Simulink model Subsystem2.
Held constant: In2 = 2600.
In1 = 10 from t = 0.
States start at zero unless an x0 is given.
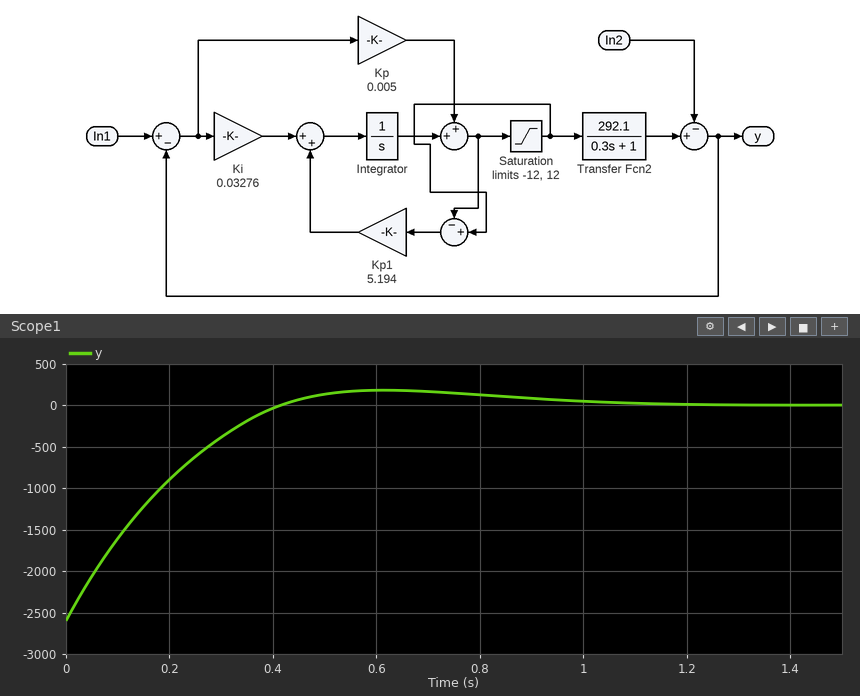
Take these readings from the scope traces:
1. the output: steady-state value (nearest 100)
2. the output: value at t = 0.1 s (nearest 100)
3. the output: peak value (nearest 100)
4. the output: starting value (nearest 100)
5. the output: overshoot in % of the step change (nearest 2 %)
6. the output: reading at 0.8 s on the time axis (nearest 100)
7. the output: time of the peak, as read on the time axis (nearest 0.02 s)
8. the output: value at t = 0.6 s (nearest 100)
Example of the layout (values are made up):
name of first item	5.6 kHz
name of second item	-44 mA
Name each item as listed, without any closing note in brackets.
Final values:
the output: steady-state value	0
the output: value at t = 0.1 s	-1600
the output: peak value	200
the output: starting value	-2600
the output: overshoot in % of the step change	6 %
the output: reading at 0.8 s on the time axis	100
the output: time of the peak, as read on the time axis	0.62 s
the output: value at t = 0.6 s	200
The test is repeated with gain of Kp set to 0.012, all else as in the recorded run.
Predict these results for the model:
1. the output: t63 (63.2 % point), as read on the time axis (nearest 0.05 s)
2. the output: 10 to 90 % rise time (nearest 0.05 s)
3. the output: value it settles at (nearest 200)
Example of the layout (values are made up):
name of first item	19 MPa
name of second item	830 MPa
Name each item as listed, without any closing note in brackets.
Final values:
the output: t63 (63.2 % point), as read on the time axis	0.20 s
the output: 10 to 90 % rise time	0.40 s
the output: value it settles at	0
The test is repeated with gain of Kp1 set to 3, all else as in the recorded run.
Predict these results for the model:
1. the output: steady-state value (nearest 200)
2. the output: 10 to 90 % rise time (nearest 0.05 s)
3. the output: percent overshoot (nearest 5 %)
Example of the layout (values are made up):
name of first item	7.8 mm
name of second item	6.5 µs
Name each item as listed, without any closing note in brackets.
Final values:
the output: steady-state value	0
the output: 10 to 90 % rise time	0.30 s
the output: percent overshoot	10 %
